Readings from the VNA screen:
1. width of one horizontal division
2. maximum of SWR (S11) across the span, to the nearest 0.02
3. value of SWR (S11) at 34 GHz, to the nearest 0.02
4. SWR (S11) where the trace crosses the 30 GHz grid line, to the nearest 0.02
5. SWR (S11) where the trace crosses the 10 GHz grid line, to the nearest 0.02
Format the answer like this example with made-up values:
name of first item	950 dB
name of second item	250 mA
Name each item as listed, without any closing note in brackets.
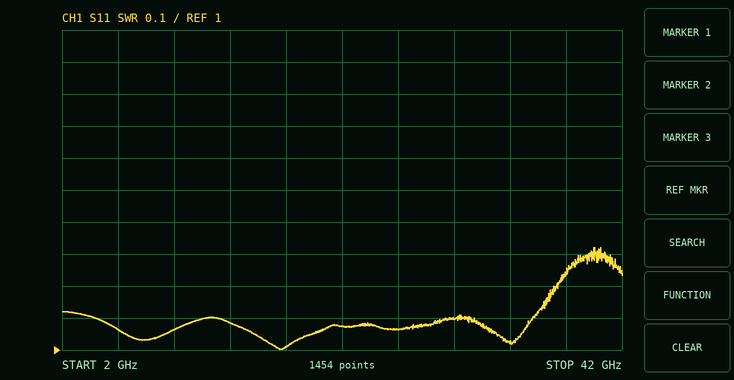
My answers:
width of one horizontal division	4 GHz
maximum of SWR (S11) across the span, to the nearest 0.02	1.32
value of SWR (S11) at 34 GHz, to the nearest 0.02	1.02
SWR (S11) where the trace crosses the 30 GHz grid line, to the nearest 0.02	1.10
SWR (S11) where the trace crosses the 10 GHz grid line, to the nearest 0.02	1.06
